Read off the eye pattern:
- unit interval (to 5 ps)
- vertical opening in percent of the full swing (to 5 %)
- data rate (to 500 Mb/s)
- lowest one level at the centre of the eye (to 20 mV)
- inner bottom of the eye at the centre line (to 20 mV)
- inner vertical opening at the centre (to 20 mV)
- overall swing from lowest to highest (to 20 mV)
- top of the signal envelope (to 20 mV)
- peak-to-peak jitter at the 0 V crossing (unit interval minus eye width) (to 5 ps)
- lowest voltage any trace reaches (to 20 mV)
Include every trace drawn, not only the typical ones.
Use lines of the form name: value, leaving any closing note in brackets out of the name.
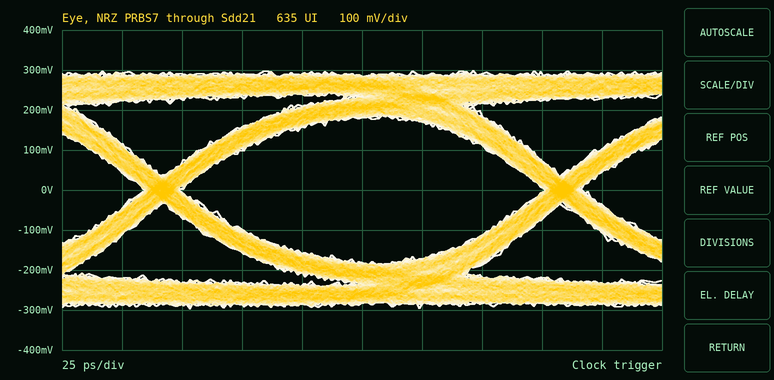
unit interval: 165 ps
vertical opening in percent of the full swing: 60 %
data rate: 6.0 Gb/s
lowest one level at the centre of the eye: 180 mV
inner bottom of the eye at the centre line: -180 mV
inner vertical opening at the centre: 360 mV
overall swing from lowest to highest: 600 mV
top of the signal envelope: 300 mV
peak-to-peak jitter at the 0 V crossing (unit interval minus eye width): 15 ps
lowest voltage any trace reaches: -300 mV
